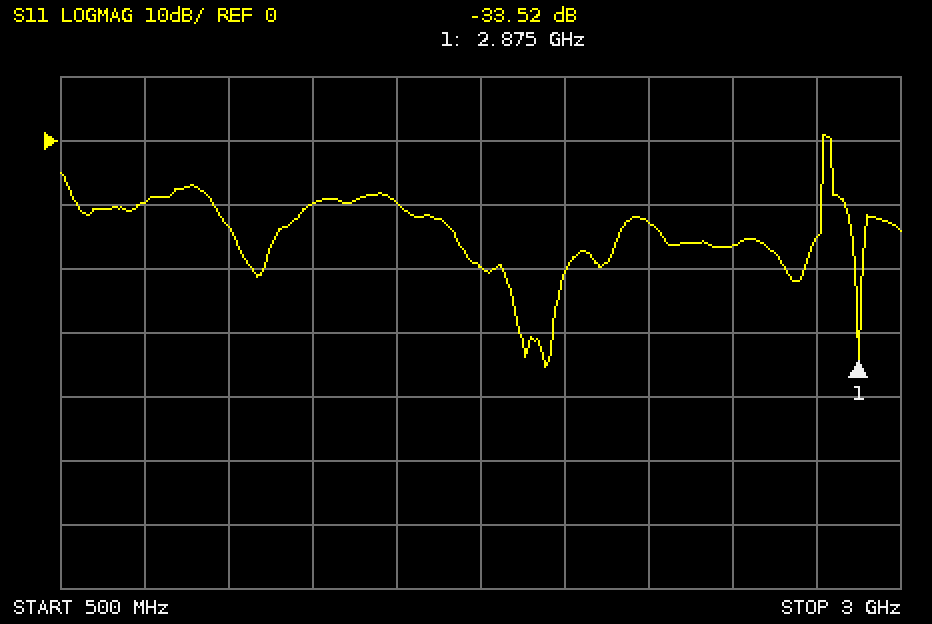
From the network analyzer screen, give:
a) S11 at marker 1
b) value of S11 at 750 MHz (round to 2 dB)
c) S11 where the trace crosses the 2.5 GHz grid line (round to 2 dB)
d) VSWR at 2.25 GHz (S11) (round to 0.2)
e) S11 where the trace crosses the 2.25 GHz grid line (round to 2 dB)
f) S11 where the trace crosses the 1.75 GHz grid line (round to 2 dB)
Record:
-33.52 dB
-10 dB
-16 dB
1.6
-12 dB
-20 dB
